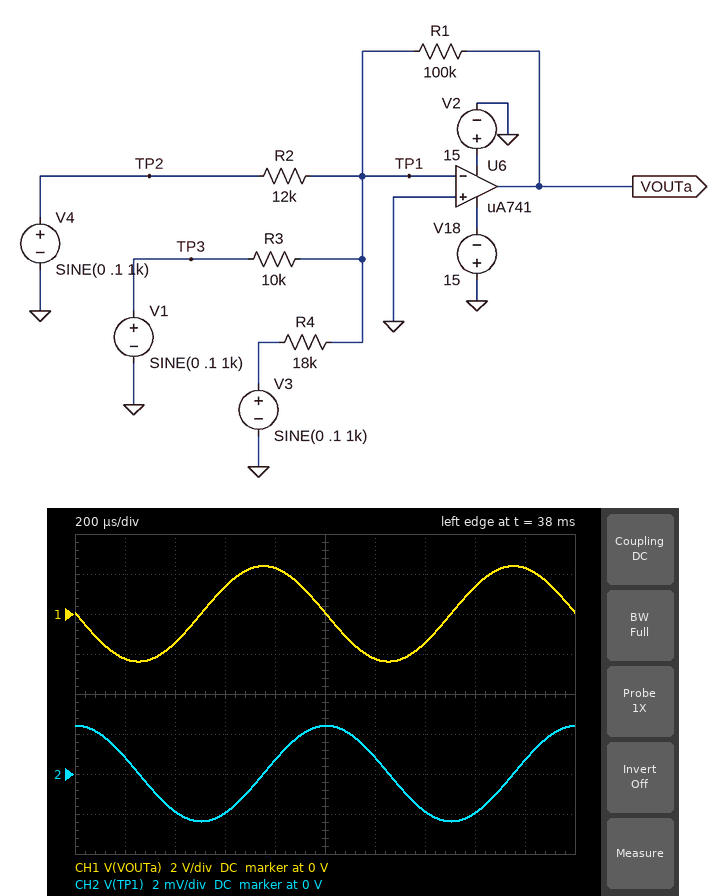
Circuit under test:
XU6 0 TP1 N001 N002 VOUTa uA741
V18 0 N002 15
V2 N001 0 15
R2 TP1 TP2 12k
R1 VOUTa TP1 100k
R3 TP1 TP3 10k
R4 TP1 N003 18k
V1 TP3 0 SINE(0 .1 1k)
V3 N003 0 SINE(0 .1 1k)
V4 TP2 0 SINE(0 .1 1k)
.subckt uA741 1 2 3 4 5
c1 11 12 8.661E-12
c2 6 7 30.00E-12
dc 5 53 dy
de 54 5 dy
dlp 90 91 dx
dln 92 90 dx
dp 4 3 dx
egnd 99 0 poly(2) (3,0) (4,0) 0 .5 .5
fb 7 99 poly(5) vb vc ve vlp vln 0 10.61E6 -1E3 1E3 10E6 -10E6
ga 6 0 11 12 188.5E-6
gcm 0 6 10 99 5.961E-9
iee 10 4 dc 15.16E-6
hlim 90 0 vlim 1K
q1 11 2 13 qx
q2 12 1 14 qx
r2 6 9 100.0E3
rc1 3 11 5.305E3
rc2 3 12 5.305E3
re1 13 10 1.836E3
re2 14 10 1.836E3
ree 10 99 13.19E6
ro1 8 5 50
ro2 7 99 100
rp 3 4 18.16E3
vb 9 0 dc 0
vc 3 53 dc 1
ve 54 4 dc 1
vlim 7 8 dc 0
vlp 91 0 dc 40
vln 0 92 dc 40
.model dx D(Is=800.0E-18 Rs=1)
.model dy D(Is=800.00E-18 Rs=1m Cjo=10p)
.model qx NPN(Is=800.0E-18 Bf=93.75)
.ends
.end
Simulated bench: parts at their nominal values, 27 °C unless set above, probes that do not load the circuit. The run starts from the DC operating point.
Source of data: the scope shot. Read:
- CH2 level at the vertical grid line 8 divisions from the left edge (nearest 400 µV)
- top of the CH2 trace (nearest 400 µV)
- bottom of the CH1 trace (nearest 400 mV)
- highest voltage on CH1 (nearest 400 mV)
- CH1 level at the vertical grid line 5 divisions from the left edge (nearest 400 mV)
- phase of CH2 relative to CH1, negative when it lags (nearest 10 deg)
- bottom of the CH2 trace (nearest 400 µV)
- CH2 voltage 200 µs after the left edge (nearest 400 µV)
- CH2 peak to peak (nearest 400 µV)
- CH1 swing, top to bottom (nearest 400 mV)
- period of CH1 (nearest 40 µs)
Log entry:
-2.0 mV
2.4 mV
-2.4 V
2.4 V
0 V
-90 deg
-2.4 mV
800 µV
4.8 mV
4.8 V
1.00 ms
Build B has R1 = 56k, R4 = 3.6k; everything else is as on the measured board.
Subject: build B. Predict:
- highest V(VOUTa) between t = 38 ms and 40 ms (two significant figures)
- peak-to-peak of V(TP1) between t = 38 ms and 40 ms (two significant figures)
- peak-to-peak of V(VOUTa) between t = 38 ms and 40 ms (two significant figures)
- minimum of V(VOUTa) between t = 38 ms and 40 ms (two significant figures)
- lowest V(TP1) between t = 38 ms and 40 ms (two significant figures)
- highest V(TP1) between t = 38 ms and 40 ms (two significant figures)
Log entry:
2.6 V
5.2 mV
5.2 V
-2.6 V
-2.6 mV
2.6 mV
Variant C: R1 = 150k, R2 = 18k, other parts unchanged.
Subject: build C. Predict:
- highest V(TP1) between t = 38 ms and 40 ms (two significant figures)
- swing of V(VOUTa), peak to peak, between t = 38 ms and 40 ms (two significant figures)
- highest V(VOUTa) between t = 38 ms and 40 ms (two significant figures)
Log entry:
3.2 mV
6.3 V
3.2 V
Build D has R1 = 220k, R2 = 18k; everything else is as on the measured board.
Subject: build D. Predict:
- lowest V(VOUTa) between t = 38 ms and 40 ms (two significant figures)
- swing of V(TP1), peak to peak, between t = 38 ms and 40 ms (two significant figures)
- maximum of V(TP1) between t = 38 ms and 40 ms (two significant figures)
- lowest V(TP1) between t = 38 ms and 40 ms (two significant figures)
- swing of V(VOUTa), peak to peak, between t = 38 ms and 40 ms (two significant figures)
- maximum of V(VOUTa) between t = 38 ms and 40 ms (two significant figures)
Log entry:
-4.6 V
9.3 mV
4.7 mV
-4.6 mV
9.3 V
4.7 V
